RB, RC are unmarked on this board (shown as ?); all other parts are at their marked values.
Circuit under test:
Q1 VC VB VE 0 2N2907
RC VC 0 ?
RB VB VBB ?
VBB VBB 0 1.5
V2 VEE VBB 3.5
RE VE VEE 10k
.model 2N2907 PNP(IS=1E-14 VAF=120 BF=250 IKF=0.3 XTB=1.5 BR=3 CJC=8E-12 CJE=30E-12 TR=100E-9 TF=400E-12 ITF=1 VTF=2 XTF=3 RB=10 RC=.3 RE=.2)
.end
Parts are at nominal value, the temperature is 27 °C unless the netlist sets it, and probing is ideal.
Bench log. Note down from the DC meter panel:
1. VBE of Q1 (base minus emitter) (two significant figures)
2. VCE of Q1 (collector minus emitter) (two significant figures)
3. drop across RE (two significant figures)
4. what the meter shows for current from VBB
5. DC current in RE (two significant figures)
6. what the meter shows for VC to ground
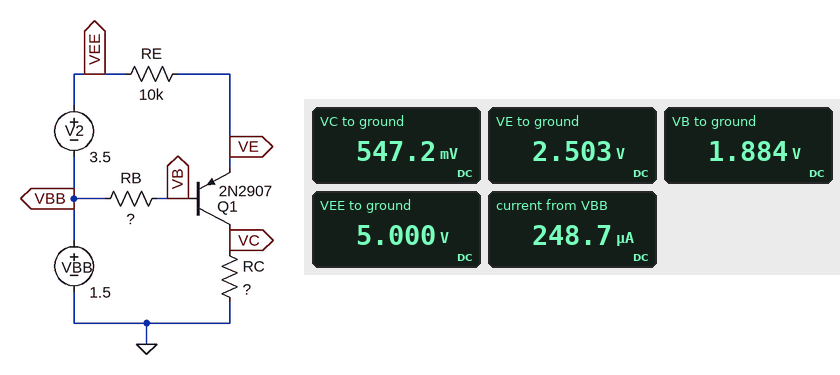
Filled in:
-620 mV
-2.0 V
2.5 V
248.7 µA
250 µA
547.2 mV
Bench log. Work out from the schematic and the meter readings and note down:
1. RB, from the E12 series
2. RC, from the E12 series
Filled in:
390 kΩ
2.2 kΩ
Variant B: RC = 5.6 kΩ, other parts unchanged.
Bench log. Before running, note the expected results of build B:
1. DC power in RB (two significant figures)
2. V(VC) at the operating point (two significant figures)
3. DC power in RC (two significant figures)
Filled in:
380 nW
1.4 V
350 µW
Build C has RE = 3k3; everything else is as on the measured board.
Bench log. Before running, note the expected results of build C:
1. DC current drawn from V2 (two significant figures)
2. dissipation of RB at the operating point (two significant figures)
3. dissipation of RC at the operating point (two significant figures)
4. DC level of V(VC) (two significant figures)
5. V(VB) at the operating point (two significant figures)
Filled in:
590 µA
2.1 µW
760 µW
1.3 V
2.4 V
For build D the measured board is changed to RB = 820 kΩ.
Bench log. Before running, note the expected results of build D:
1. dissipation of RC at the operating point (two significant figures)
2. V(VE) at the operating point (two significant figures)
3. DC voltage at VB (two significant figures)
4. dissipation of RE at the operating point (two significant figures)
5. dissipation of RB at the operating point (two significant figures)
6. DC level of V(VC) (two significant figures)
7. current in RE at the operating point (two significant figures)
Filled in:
100 µW
2.8 V
2.2 V
480 µW
600 nW
480 mV
220 µA
